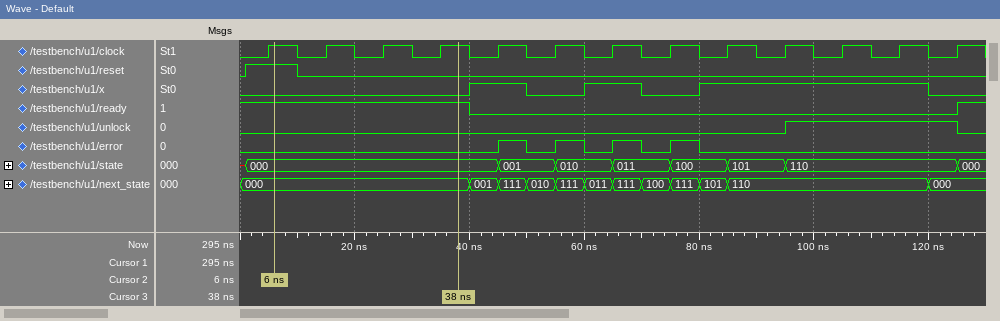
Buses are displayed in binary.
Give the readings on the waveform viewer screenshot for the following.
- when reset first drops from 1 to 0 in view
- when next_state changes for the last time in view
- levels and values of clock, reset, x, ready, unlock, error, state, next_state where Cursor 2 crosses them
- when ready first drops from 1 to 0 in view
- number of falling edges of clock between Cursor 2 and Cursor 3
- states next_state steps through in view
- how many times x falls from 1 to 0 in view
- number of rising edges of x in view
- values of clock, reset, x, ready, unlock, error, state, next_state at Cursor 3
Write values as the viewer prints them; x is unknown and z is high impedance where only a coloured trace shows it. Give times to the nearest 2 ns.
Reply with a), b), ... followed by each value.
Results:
a) 10 ns
b) 120 ns
c) clock=1, reset=1, x=0, ready=1, unlock=0, error=0, state=000, next_state=000
d) 40 ns
e) 3
f) 000, 001, 111, 010, 111, 011, 111, 100, 111, 101, 110, 000
g) 3
h) 3
i) clock=1, reset=0, x=0, ready=1, unlock=0, error=0, state=000, next_state=000
